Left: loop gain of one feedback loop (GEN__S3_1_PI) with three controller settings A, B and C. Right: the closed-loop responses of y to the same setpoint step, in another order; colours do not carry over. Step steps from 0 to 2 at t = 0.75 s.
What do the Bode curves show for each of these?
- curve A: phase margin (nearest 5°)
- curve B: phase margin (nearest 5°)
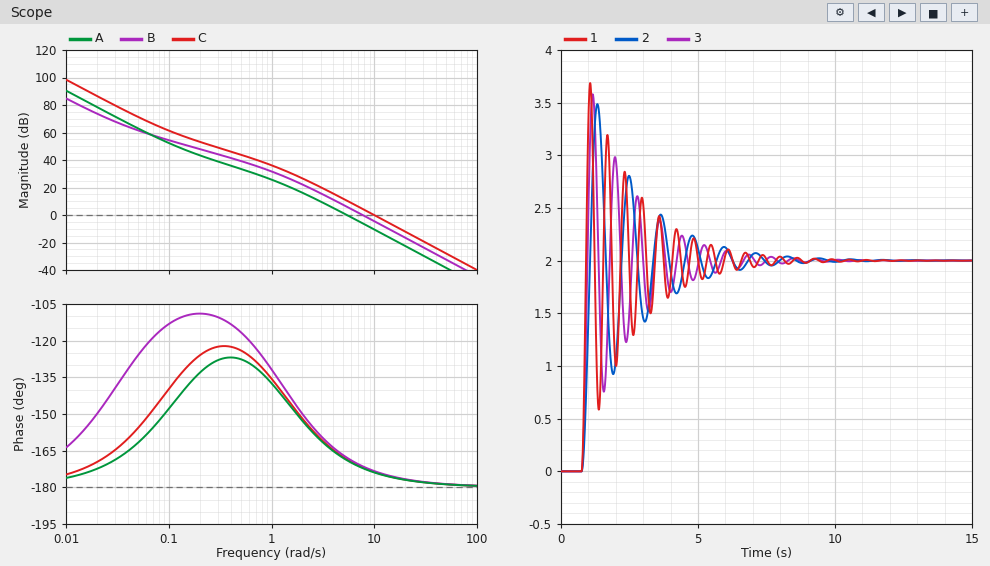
10°
10°
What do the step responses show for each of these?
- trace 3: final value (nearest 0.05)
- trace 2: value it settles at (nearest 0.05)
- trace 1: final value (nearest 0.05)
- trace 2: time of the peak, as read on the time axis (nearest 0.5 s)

2.00
2.00
2.00
1.5 s
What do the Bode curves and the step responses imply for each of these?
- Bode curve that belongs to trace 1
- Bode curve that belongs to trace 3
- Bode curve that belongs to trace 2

C
B
A
